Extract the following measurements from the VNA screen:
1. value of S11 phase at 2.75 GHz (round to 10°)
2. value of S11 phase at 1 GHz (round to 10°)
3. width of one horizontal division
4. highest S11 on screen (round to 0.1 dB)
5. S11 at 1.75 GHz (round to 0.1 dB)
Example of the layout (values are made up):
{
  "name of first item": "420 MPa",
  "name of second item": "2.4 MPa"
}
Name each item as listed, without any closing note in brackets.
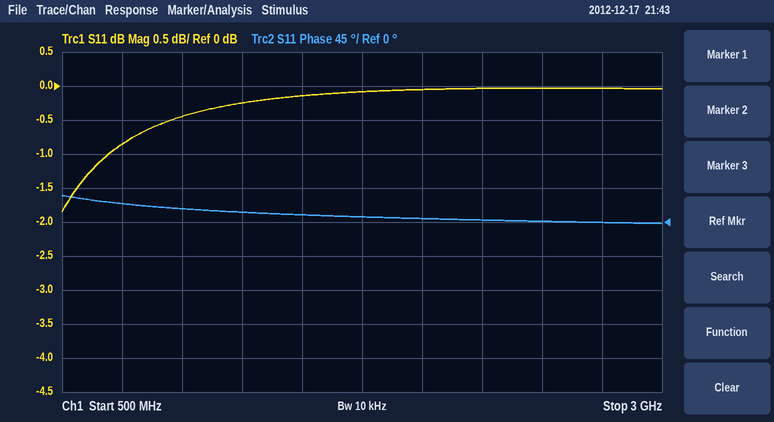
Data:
{
  "value of S11 phase at 2.75 GHz": "0°",
  "value of S11 phase at 1 GHz": "20°",
  "width of one horizontal division": "250 MHz",
  "highest S11 on screen": "0.0 dB",
  "S11 at 1.75 GHz": "-0.1 dB"
}
